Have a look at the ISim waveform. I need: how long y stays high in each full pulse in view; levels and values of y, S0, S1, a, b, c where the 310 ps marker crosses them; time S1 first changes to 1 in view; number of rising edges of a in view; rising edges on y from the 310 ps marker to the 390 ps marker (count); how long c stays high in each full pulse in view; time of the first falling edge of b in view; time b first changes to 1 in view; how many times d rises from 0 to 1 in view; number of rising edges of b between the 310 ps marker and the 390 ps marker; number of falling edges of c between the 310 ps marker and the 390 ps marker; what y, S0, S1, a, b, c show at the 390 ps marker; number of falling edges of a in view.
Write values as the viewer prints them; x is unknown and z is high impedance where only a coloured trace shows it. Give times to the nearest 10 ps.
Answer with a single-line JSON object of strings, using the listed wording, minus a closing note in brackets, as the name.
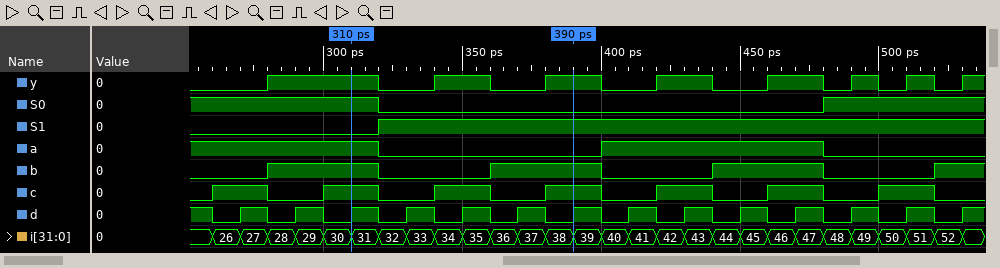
{"how long y stays high in each full pulse in view": "40 ps, 20 ps, 20 ps, 20 ps, 20 ps, 10 ps, 10 ps", "levels and values of y, S0, S1, a, b, c where the 310 ps marker crosses them": "y=1, S0=1, S1=0, a=1, b=1, c=1", "time S1 first changes to 1 in view": "320 ps", "number of rising edges of a in view": "1", "rising edges on y from the 310 ps marker to the 390 ps marker": "2", "how long c stays high in each full pulse in view": "20 ps, 20 ps, 20 ps, 20 ps, 20 ps, 20 ps, 20 ps", "time of the first falling edge of b in view": "320 ps", "time b first changes to 1 in view": "280 ps", "how many times d rises from 0 to 1 in view": "14", "number of rising edges of b between the 310 ps marker and the 390 ps marker": "1", "number of falling edges of c between the 310 ps marker and the 390 ps marker": "2", "what y, S0, S1, a, b, c show at the 390 ps marker": "y=1, S0=0, S1=1, a=0, b=1, c=1", "number of falling edges of a in view": "2"}
